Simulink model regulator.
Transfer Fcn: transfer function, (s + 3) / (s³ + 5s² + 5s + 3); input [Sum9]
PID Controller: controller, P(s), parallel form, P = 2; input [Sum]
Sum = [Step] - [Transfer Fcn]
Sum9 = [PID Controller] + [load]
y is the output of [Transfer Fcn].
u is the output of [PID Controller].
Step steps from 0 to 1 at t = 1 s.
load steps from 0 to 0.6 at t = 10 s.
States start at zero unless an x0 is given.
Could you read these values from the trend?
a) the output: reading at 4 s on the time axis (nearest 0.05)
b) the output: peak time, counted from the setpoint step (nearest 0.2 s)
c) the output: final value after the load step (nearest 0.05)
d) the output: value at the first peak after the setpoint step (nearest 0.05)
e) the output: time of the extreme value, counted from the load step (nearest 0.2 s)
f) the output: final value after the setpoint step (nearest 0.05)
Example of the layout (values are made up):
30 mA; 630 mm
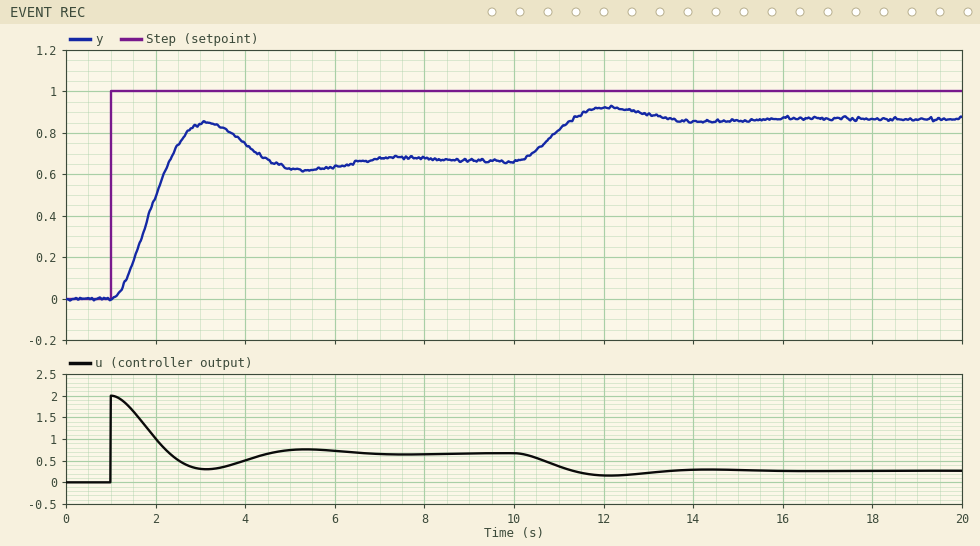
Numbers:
0.75; 2.2 s; 0.85; 0.85; 2.2 s; 0.65
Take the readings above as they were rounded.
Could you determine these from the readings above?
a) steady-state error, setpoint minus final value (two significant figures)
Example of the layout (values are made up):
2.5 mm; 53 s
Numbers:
0.35
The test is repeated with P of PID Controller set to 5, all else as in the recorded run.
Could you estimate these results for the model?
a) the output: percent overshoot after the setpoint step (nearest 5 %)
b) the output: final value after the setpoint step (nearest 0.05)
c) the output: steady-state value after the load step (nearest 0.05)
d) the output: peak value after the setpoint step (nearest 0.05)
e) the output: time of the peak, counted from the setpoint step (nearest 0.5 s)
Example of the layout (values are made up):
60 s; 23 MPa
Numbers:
40 %; 0.85; 0.95; 1.15; 1.5 s
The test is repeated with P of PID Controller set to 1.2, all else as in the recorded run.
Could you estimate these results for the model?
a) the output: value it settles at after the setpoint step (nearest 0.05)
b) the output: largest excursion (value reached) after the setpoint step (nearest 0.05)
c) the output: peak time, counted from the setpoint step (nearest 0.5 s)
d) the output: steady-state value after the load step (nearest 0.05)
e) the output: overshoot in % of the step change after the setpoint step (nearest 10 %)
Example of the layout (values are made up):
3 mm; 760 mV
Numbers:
0.55; 0.65; 2.5 s; 0.80; 20 %
